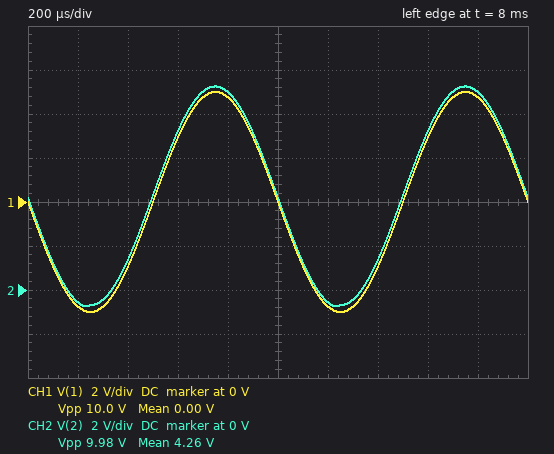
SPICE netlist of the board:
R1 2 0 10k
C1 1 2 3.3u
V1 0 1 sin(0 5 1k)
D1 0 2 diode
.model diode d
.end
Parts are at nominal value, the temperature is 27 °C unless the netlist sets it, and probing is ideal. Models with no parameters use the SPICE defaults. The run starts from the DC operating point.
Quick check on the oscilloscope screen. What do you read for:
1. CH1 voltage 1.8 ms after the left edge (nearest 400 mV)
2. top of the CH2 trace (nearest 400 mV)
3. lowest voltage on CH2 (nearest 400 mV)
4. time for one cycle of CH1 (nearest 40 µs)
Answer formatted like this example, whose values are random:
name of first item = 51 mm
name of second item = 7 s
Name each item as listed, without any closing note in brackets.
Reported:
CH1 voltage 1.8 ms after the left edge = 4.8 V
top of the CH2 trace = 9.2 V
lowest voltage on CH2 = -800 mV
time for one cycle of CH1 = 1.00 ms
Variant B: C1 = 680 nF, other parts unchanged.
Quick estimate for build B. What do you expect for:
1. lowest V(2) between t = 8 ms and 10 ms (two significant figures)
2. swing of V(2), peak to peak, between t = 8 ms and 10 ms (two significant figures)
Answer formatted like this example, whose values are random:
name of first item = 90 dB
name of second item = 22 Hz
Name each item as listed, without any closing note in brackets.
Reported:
lowest V(2) between t = 8 ms and 10 ms = -710 mV
swing of V(2), peak to peak, between t = 8 ms and 10 ms = 9.8 V
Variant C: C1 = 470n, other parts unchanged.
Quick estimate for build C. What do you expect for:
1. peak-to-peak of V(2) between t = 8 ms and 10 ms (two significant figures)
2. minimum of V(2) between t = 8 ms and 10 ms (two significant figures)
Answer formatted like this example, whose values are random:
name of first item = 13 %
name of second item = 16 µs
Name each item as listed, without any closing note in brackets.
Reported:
peak-to-peak of V(2) between t = 8 ms and 10 ms = 9.6 V
minimum of V(2) between t = 8 ms and 10 ms = -710 mV
